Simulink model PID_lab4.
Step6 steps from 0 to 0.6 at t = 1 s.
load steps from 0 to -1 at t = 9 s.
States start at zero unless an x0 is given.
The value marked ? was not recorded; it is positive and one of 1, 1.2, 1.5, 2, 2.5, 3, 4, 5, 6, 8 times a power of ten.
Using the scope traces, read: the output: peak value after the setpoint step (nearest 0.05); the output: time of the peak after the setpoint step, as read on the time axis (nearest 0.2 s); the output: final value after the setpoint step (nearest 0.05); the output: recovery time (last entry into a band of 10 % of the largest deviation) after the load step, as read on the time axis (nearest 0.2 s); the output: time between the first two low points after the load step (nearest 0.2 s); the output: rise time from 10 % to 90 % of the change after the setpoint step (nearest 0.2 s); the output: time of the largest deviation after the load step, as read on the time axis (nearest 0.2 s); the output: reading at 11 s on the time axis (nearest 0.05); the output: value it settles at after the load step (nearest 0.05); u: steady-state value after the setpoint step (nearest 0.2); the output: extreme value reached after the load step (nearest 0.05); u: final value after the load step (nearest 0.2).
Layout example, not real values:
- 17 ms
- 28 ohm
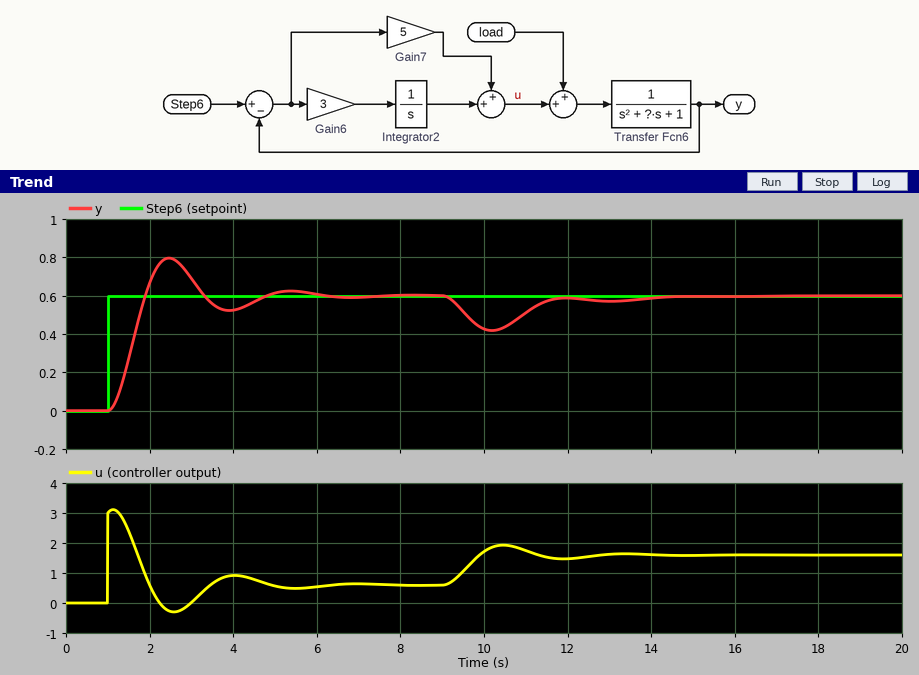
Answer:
- 0.80
- 2.4 s
- 0.60
- 13.8 s
- 2.8 s
- 0.6 s
- 10.2 s
- 0.50
- 0.60
- 0.6
- 0.40
- 1.6
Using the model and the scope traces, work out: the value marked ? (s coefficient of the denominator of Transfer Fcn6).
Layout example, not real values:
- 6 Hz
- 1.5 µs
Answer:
- 2
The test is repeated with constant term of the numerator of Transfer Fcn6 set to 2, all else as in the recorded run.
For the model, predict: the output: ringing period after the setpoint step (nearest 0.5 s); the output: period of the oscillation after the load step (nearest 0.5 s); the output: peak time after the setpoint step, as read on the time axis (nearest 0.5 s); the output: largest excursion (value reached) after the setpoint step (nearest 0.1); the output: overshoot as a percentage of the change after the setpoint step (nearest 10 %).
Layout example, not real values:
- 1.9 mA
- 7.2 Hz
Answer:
- 2.0 s
- 2.0 s
- 2.0 s
- 0.9
- 50 %
